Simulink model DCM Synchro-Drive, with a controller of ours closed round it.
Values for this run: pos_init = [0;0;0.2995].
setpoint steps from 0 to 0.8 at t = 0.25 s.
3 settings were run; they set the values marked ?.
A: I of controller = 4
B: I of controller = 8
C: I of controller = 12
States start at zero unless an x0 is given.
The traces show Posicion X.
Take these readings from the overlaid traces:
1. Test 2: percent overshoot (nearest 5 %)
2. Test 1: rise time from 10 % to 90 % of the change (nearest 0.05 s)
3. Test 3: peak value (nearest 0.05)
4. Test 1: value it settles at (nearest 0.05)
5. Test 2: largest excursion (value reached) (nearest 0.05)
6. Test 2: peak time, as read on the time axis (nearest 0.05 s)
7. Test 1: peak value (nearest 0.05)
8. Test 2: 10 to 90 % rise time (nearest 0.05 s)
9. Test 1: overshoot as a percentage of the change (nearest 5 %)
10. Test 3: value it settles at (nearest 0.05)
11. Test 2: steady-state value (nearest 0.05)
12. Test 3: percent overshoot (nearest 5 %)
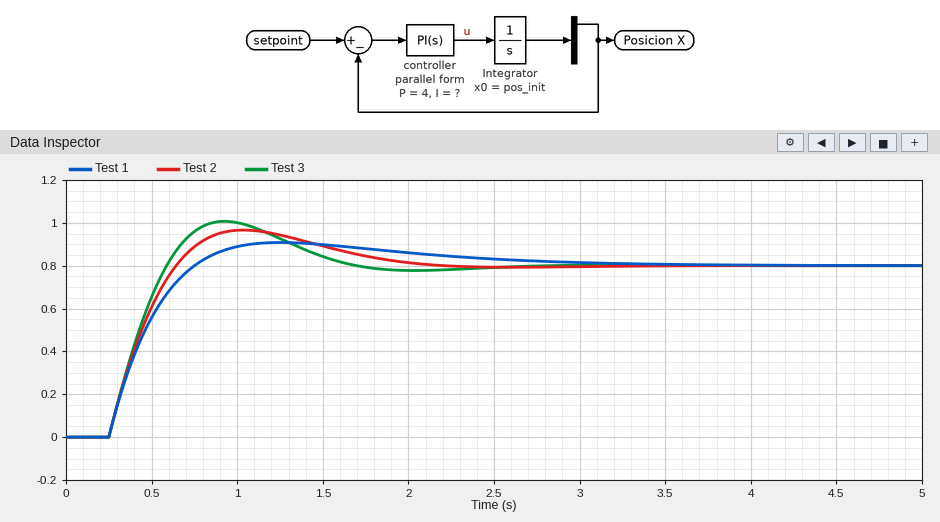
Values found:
20 %
0.35 s
1.00
0.80
0.95
1.05 s
0.90
0.30 s
15 %
0.80
0.80
25 %
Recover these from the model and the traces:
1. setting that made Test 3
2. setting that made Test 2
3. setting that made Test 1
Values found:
C
B
A
